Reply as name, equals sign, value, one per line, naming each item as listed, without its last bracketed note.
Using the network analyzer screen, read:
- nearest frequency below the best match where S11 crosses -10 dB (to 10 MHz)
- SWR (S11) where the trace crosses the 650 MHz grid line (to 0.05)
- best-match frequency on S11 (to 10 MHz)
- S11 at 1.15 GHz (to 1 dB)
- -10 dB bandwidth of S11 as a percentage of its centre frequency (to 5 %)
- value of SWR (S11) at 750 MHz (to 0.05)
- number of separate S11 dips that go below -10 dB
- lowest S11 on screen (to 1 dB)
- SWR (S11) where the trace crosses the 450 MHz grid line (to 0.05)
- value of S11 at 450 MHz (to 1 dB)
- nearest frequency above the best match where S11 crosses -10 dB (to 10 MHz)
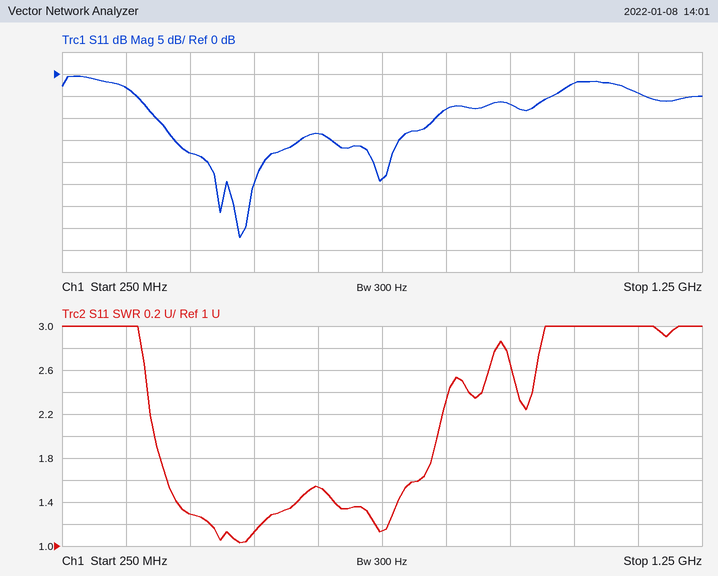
nearest frequency below the best match where S11 crosses -10 dB = 400 MHz
SWR (S11) where the trace crosses the 650 MHz grid line = 1.55
best-match frequency on S11 = 530 MHz
S11 at 1.15 GHz = -4 dB
-10 dB bandwidth of S11 as a percentage of its centre frequency = 70 %
value of SWR (S11) at 750 MHz = 1.15
number of separate S11 dips that go below -10 dB = 3
lowest S11 on screen = -37 dB
SWR (S11) where the trace crosses the 450 MHz grid line = 1.30
value of S11 at 450 MHz = -18 dB
nearest frequency above the best match where S11 crosses -10 dB = 830 MHz
